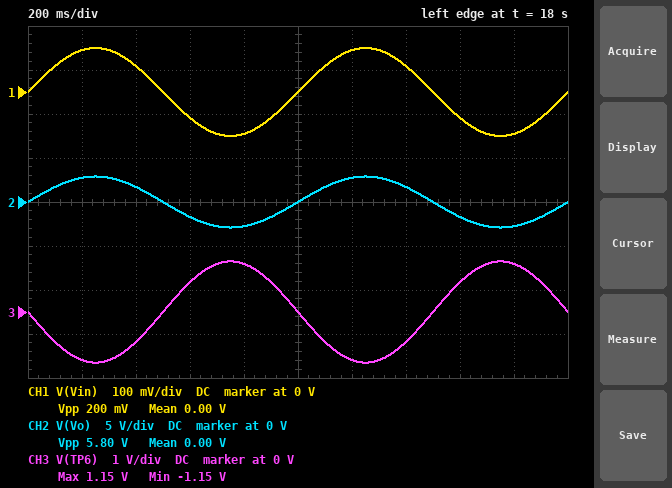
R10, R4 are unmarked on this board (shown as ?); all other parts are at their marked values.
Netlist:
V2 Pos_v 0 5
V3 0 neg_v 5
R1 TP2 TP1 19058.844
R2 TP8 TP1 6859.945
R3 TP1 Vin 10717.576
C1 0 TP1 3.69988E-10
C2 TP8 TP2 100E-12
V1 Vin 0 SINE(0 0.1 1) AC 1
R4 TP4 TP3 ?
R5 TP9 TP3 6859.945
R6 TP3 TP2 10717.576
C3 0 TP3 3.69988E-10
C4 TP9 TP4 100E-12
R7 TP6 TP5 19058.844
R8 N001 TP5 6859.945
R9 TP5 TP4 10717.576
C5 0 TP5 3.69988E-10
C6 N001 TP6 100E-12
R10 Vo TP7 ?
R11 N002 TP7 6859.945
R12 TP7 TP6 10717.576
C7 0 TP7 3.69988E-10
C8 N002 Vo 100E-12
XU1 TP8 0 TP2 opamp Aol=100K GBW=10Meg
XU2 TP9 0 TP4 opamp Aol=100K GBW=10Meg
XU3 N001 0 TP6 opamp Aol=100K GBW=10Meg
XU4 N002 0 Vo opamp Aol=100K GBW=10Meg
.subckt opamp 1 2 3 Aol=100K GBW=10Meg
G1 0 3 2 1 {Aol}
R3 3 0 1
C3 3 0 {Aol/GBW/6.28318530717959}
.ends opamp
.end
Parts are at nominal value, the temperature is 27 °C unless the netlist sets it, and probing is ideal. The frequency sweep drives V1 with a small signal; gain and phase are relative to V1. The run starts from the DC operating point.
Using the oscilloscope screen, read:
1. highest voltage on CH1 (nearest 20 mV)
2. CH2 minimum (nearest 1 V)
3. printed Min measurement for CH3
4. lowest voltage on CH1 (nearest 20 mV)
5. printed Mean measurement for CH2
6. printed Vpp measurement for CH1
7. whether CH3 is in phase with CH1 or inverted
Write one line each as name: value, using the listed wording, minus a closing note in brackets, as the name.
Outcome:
highest voltage on CH1: 100 mV
CH2 minimum: -3 V
printed Min measurement for CH3: -1.15 V
lowest voltage on CH1: -100 mV
printed Mean measurement for CH2: 0.00 V
printed Vpp measurement for CH1: 200 mV
whether CH3 is in phase with CH1 or inverted: inverted
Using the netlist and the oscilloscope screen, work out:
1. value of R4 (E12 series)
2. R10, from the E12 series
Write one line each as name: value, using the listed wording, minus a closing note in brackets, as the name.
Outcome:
value of R4: 39 kΩ
R10, from the E12 series: 27 kΩ
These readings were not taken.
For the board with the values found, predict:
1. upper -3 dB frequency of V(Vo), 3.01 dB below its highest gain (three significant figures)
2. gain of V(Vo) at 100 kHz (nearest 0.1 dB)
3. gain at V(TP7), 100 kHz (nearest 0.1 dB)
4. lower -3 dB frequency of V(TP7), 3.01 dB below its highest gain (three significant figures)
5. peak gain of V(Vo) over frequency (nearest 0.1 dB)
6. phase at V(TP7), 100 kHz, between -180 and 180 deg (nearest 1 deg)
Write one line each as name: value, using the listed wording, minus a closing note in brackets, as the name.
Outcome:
upper -3 dB frequency of V(Vo), 3.01 dB below its highest gain: 19.0 kHz
gain of V(Vo) at 100 kHz: -13.3 dB
gain at V(TP7), 100 kHz: -20.4 dB
lower -3 dB frequency of V(TP7), 3.01 dB below its highest gain: 11.4 kHz
peak gain of V(Vo) over frequency: 29.2 dB
phase at V(TP7), 100 kHz, between -180 and 180 deg: 163 deg
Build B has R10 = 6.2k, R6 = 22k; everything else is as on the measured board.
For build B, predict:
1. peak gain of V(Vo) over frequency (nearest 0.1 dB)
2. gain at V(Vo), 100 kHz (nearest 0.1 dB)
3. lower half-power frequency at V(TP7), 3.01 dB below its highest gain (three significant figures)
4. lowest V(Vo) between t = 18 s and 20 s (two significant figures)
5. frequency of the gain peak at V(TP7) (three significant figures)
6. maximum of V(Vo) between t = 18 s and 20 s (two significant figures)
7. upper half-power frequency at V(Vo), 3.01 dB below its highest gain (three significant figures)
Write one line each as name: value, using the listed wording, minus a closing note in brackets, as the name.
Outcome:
peak gain of V(Vo) over frequency: 10.2 dB
gain at V(Vo), 100 kHz: -21.0 dB
lower half-power frequency at V(TP7), 3.01 dB below its highest gain: 15.7 kHz
lowest V(Vo) between t = 18 s and 20 s: -320 mV
frequency of the gain peak at V(TP7): 32.7 kHz
maximum of V(Vo) between t = 18 s and 20 s: 320 mV
upper half-power frequency at V(Vo), 3.01 dB below its highest gain: 27.2 kHz
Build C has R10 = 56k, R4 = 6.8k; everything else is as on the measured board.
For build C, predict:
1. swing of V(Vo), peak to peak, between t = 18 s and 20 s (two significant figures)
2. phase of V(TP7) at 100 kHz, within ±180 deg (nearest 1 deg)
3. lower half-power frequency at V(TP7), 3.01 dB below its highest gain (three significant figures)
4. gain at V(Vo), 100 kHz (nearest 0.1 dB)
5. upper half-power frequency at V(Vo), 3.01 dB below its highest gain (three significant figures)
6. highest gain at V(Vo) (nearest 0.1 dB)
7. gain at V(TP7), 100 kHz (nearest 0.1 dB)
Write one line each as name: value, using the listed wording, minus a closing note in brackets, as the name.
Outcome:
swing of V(Vo), peak to peak, between t = 18 s and 20 s: 2.1 V
phase of V(TP7) at 100 kHz, within ±180 deg: -157 deg
lower half-power frequency at V(TP7), 3.01 dB below its highest gain: 10.9 kHz
gain at V(Vo), 100 kHz: -15.5 dB
upper half-power frequency at V(Vo), 3.01 dB below its highest gain: 16.7 kHz
highest gain at V(Vo): 20.4 dB
gain at V(TP7), 100 kHz: -22.6 dB
